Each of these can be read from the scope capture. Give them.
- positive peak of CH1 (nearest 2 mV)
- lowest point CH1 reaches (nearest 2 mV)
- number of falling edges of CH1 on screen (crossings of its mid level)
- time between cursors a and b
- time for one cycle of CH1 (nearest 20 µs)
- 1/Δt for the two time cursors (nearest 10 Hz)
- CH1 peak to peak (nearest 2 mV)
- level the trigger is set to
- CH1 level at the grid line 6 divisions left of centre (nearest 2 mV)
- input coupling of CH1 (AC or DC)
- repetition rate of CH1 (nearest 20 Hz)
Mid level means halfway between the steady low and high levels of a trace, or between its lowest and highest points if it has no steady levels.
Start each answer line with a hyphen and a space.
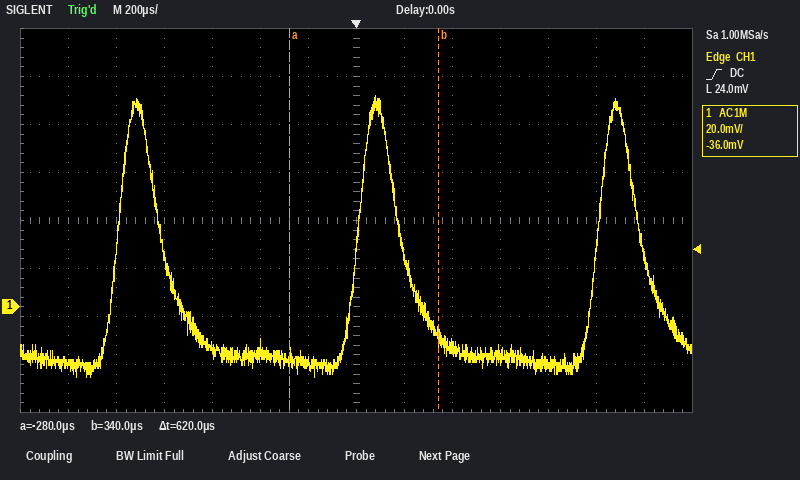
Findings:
- 88 mV
- -30 mV
- 3
- 620 µs
- 1.00 ms
- 1.61 kHz
- 118 mV
- 24.0 mV
- -24 mV
- AC
- 1.00 kHz
